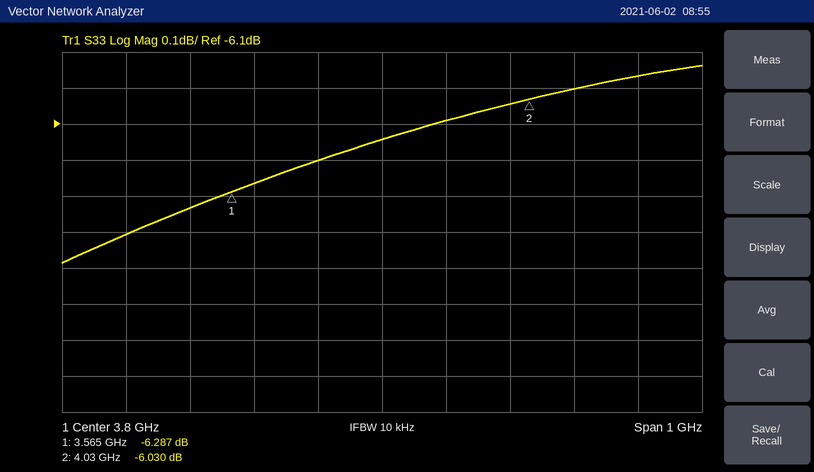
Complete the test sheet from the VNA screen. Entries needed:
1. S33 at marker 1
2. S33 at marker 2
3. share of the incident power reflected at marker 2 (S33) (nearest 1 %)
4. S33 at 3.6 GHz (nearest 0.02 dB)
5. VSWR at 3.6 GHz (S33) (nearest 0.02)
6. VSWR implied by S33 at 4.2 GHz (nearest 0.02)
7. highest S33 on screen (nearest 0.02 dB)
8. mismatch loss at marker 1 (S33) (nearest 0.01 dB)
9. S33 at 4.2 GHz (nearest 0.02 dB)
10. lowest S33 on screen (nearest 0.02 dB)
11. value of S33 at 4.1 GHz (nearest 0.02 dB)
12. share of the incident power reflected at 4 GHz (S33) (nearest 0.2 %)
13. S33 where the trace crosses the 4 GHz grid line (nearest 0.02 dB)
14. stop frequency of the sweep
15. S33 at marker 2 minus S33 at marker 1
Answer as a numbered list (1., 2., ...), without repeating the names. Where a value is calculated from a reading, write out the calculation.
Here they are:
1. -6.287 dB
2. -6.030 dB
3. 10^(-6.03/10) ≈ 25 %
4. -6.26 dB
5. |Γ| = 10^(-6.26/20) = 0.4864; VSWR = (1 + 0.4864)/(1 − 0.4864) ≈ 2.89, so 2.90 to the nearest 0.02
6. |Γ| = 10^(-5.96/20) = 0.5035; VSWR = (1 + 0.5035)/(1 − 0.5035) ≈ 3.03, so 3.02 to the nearest 0.02
7. -5.94 dB
8. −10 log10(1 − 10^(-6.287/10)) ≈ 1.16 dB
9. -5.96 dB
10. -6.48 dB
11. -6.00 dB
12. 10^(-6.04/10) ≈ 24.9 %, so 24.8 % to the nearest 0.2 %
13. -6.04 dB
14. 4.3 GHz
15. -6.03 − (-6.287) = 0.257 dB
